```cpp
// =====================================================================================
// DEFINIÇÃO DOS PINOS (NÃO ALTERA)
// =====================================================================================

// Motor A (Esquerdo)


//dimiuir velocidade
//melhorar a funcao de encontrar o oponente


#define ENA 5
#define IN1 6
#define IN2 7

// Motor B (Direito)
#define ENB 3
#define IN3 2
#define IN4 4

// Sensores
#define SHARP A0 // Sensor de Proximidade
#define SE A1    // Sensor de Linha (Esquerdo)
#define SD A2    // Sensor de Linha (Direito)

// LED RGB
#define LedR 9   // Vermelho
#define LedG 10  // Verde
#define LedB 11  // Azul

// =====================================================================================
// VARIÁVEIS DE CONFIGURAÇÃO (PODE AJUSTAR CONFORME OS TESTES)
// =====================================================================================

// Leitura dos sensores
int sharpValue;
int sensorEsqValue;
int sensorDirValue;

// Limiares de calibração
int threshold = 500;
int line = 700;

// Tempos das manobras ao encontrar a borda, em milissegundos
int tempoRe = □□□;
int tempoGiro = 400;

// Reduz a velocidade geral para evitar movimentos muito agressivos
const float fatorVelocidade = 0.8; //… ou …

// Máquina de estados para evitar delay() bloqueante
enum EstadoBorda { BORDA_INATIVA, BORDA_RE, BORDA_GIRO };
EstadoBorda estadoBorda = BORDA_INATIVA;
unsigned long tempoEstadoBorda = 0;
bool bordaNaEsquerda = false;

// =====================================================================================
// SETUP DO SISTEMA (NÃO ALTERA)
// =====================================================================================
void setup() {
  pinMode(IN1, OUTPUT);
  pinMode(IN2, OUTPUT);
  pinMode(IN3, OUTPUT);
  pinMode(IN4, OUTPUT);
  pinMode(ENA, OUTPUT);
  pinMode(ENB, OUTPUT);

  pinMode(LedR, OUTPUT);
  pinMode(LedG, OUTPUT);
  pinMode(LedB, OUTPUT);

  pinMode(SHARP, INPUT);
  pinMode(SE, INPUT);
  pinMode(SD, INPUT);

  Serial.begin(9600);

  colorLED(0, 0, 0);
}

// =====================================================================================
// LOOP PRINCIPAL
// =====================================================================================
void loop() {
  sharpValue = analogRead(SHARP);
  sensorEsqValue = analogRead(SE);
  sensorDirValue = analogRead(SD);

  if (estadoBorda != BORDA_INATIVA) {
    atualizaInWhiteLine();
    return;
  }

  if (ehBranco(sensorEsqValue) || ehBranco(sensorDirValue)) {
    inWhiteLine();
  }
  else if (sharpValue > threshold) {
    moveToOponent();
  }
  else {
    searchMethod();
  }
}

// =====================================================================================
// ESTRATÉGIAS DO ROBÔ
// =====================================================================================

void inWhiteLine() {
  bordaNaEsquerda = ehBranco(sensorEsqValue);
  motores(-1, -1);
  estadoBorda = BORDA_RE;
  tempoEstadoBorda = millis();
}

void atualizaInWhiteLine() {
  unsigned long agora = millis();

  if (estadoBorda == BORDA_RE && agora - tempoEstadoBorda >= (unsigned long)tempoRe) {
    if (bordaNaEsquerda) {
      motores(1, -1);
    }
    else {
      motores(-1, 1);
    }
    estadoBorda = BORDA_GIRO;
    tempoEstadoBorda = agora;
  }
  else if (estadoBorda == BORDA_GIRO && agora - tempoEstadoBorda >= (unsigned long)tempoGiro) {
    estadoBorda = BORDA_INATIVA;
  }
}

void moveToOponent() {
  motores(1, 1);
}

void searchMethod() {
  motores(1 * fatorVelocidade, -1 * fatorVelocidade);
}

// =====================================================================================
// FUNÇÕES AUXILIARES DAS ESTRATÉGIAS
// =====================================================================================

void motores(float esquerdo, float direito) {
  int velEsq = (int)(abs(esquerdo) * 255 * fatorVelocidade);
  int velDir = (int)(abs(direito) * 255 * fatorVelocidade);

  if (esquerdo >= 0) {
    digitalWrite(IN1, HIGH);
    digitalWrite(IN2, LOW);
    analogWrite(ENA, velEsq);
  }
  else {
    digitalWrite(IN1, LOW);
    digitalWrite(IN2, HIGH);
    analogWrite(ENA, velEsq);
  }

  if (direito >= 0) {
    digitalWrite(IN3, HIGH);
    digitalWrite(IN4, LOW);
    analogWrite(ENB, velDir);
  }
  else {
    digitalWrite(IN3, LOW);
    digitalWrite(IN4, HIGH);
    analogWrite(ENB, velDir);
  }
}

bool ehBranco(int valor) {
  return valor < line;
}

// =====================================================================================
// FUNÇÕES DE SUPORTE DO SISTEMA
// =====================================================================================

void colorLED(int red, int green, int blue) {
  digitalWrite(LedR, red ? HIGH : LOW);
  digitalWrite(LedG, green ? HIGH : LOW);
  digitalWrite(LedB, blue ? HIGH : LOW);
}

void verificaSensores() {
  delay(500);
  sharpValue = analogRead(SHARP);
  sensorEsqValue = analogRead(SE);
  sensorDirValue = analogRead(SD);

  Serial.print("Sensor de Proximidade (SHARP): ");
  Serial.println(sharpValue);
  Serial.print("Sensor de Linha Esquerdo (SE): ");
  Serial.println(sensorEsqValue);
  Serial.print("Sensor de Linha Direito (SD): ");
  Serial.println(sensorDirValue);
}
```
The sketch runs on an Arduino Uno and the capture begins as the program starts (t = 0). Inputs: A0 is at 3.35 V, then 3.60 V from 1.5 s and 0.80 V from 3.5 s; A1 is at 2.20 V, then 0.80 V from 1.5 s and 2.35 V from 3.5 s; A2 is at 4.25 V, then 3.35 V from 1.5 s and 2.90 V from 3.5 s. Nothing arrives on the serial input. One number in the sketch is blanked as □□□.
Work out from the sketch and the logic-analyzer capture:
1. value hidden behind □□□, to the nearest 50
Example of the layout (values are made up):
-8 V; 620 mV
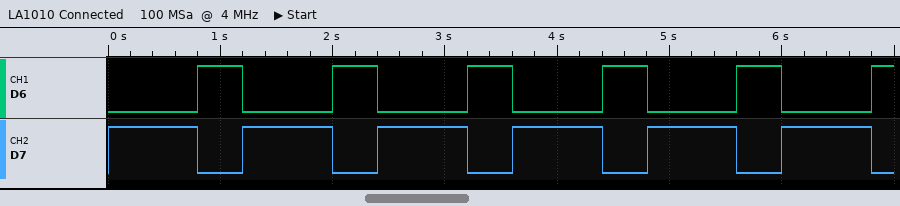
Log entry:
800
